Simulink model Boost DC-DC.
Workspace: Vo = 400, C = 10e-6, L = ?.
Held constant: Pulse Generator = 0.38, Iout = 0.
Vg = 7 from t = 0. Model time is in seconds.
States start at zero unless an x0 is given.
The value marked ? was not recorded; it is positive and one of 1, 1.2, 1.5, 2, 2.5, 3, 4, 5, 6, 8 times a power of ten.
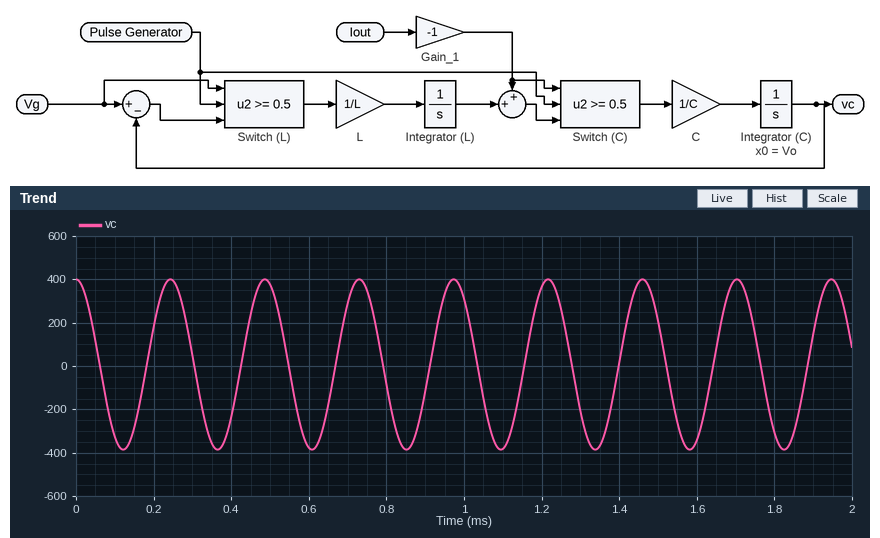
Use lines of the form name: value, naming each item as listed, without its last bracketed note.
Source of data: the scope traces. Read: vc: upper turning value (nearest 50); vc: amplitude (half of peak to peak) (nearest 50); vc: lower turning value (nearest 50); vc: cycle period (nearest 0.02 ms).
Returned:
vc: upper turning value: 400
vc: amplitude (half of peak to peak): 400
vc: lower turning value: -400
vc: cycle period: 0.24 ms
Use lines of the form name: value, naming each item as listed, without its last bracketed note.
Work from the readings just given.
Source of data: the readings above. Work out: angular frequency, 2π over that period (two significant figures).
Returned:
angular frequency, 2π over that period: 26 rad/ms
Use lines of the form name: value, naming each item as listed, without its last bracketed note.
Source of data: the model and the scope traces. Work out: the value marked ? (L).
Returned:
the value marked ?: 0.00015
